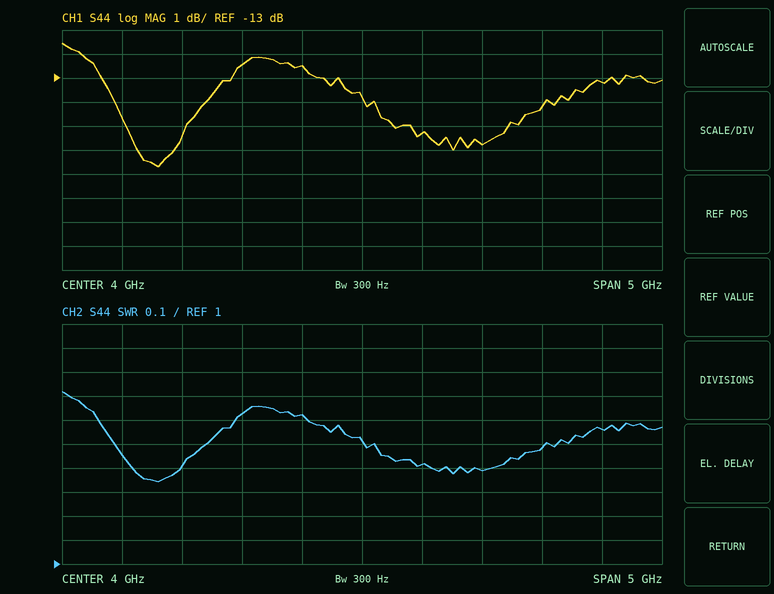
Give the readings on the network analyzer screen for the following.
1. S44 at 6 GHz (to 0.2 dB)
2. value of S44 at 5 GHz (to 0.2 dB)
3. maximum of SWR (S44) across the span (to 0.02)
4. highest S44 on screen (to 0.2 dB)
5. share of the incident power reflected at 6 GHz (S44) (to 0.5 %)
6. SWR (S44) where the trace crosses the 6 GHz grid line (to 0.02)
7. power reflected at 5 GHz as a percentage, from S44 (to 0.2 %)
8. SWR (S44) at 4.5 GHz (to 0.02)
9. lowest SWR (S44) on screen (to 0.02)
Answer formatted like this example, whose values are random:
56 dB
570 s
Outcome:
-13.2 dB
-15.8 dB
1.72
-11.6 dB
5.0 %
1.56
2.6 %
1.42
1.34
